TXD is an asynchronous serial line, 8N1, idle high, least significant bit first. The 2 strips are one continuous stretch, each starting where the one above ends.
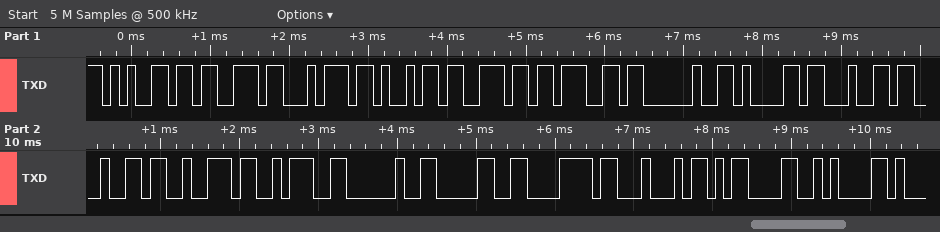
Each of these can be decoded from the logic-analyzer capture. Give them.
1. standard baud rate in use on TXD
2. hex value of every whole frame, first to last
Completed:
9600 baud
0x65 0x73 0x74 0x69 0x6E 0x67 0x20 0x61 0x64 0x64 0x72 0x3A 0x20 0x30 0x78 0x44 0x0D 0x0A
